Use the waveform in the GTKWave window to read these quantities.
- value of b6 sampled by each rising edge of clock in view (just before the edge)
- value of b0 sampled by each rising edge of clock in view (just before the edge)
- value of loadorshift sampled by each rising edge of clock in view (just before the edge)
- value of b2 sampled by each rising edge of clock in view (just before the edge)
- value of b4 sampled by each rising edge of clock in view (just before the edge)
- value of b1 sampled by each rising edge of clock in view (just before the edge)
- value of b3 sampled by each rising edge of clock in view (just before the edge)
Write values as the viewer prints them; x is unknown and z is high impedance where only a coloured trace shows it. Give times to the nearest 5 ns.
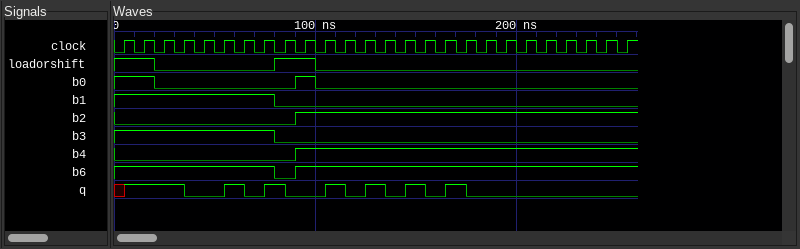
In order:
1 1 1 1 1 1 1 1 0 1 1 1 1 1 1 1 1 1 1 1 1 1 1 1 1 1
1 1 0 0 0 0 0 0 0 1 0 0 0 0 0 0 0 0 0 0 0 0 0 0 0 0
1 1 0 0 0 0 0 0 1 1 0 0 0 0 0 0 0 0 0 0 0 0 0 0 0 0
0 0 0 0 0 0 0 0 0 1 1 1 1 1 1 1 1 1 1 1 1 1 1 1 1 1
0 0 0 0 0 0 0 0 0 1 1 1 1 1 1 1 1 1 1 1 1 1 1 1 1 1
1 1 1 1 1 1 1 1 0 0 0 0 0 0 0 0 0 0 0 0 0 0 0 0 0 0
1 1 1 1 1 1 1 1 0 0 0 0 0 0 0 0 0 0 0 0 0 0 0 0 0 0
